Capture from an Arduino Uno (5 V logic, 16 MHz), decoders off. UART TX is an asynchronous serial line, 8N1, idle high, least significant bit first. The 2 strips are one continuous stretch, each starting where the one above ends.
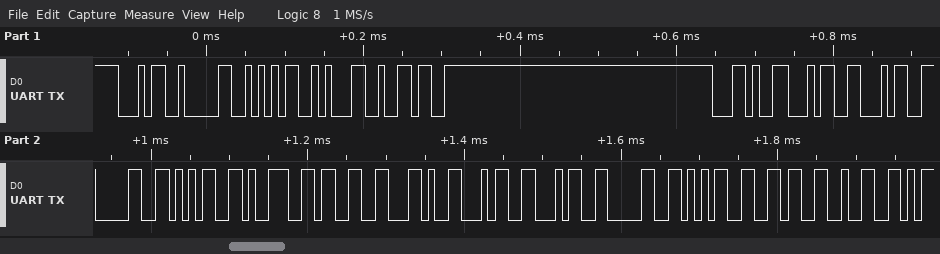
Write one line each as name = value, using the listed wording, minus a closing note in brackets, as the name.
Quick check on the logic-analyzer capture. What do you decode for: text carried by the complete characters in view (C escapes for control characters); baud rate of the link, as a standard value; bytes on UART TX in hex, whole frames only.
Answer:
text carried by the complete characters in view = "40516,440593,440562"
baud rate of the link, as a standard value = 115200 baud
bytes on UART TX in hex, whole frames only = 34 30 35 31 36 2C 34 34 30 35 39 33 2C 34 34 30 35 36 32
